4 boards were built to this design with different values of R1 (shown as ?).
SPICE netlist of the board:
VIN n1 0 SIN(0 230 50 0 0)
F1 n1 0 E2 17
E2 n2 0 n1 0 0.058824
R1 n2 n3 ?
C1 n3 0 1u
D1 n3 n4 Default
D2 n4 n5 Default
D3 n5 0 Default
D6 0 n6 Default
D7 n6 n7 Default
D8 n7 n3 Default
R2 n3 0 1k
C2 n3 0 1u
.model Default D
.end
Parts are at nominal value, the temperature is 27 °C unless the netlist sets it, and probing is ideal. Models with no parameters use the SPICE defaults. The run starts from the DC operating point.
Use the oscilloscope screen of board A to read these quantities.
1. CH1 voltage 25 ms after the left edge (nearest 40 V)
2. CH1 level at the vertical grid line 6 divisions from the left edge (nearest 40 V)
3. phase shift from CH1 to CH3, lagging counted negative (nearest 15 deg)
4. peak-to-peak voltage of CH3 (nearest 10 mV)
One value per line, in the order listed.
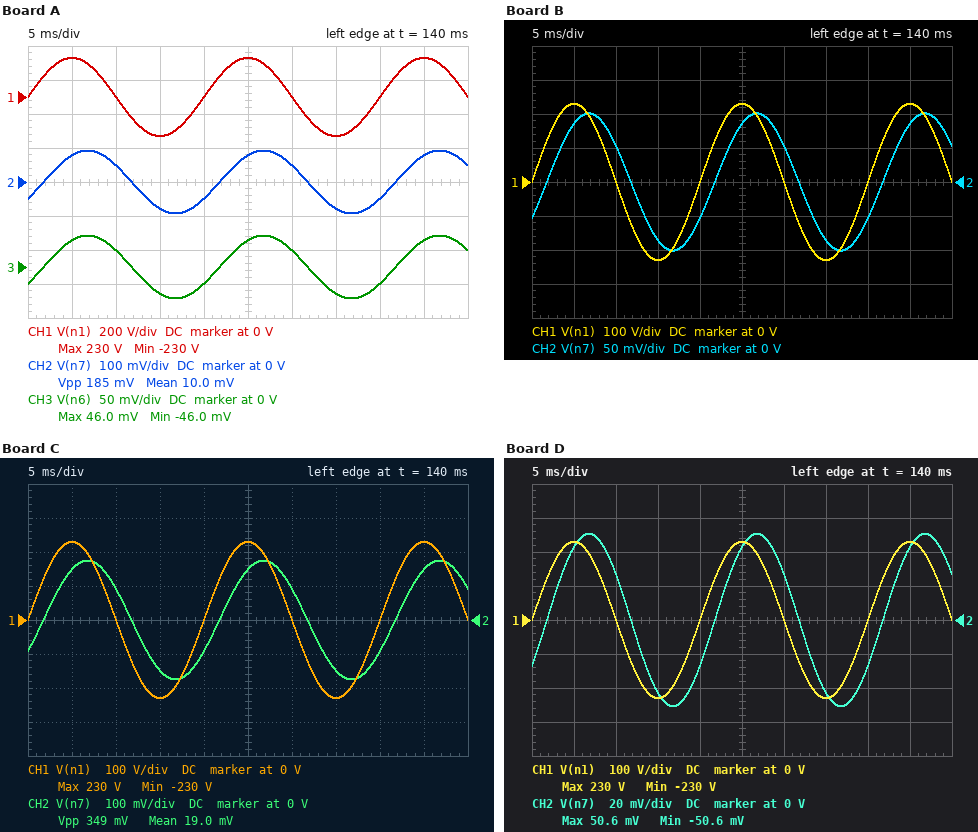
240 V
0 V
-30 deg
90 mV
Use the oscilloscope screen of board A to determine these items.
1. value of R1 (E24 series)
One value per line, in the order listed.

82 kΩ
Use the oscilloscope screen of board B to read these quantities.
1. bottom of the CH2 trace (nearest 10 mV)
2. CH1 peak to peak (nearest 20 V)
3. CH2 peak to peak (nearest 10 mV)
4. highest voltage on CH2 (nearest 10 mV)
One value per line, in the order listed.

-100 mV
460 V
200 mV
100 mV
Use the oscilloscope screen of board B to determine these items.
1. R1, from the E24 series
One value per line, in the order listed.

75 kΩ
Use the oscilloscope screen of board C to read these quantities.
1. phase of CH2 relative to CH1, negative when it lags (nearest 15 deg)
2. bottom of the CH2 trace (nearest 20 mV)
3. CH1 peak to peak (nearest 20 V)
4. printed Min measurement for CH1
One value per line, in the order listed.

-30 deg
-180 mV
460 V
-230 V
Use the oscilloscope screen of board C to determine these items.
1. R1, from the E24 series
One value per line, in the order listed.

43 kΩ
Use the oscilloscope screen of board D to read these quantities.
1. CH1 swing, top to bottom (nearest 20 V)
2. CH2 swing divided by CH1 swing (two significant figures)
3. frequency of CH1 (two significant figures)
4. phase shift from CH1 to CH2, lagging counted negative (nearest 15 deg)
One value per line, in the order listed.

460 V
0.00022
50 Hz
-30 deg
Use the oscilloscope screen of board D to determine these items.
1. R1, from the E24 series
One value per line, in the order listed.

150 kΩ
